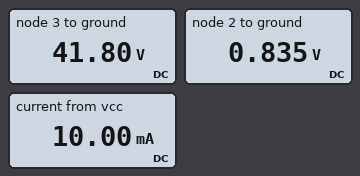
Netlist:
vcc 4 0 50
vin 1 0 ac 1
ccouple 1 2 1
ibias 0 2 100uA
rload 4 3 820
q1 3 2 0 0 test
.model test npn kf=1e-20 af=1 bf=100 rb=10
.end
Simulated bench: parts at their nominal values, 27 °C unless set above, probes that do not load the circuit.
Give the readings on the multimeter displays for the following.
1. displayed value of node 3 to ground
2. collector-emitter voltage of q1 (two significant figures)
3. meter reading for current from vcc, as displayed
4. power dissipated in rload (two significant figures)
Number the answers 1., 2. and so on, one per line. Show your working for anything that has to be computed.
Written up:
1. 41.80 V
2. 41.8 V = 42 V
3. 10.00 mA
4. (50 V - 41.8 V)^2 / 820 Ω = 82 mW
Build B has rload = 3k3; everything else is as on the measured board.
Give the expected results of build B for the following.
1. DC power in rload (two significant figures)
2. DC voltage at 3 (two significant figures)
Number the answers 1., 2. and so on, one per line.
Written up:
1. 330 mW
2. 17 V
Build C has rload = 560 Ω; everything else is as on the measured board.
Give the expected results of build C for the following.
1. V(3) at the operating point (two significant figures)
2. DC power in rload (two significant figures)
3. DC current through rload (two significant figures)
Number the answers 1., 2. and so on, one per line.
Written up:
1. 44 V
2. 56 mW
3. 10 mA
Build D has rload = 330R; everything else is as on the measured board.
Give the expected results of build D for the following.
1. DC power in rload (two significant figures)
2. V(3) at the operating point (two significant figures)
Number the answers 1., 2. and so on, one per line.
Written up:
1. 33 mW
2. 47 V
